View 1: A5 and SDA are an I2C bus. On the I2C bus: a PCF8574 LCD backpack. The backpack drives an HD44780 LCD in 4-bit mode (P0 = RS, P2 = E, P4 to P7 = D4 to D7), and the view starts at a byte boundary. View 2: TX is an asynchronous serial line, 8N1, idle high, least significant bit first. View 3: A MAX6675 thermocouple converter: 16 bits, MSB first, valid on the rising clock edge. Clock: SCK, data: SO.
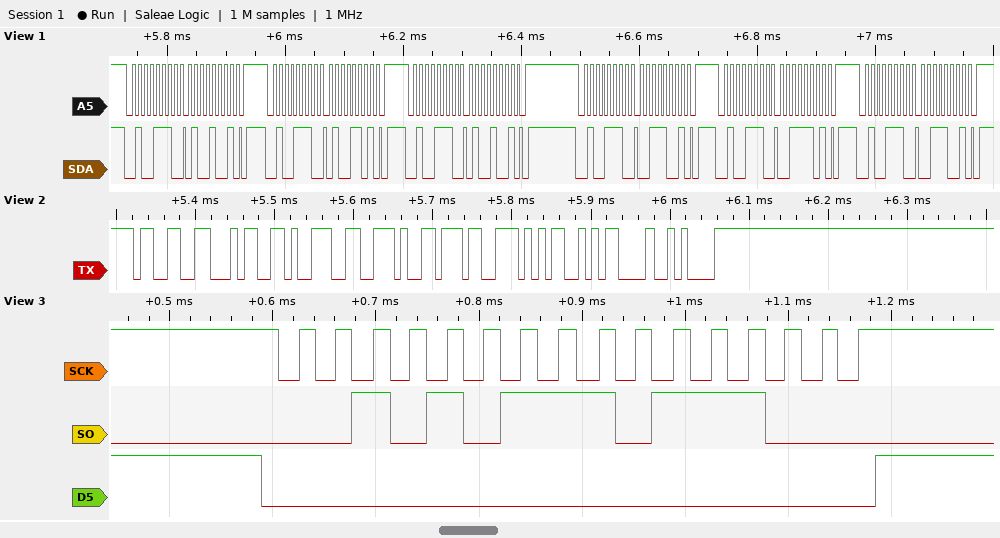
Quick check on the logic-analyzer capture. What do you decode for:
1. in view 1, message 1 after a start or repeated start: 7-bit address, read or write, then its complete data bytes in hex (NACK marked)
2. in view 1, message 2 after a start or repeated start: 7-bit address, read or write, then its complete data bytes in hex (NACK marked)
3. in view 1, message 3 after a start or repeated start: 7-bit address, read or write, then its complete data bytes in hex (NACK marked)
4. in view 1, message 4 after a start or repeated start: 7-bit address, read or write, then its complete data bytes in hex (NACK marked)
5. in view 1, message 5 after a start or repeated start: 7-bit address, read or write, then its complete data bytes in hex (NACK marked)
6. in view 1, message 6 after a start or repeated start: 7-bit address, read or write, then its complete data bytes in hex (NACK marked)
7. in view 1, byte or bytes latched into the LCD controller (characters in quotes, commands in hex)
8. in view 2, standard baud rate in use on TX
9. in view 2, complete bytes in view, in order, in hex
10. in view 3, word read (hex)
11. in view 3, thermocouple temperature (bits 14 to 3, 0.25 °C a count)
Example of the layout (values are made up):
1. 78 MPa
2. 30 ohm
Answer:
1. 0x27 write: 49
2. 0x27 write: 4D
3. 0x27 write: 49
4. 0x27 write: 39
5. 0x27 write: 3D
6. 0x27 write: 39
7. 'C'
8. 115200 baud
9. 33 34 39 2E 37 35 0D 0A
10. 0x2BB8
11. 349.75 °C
